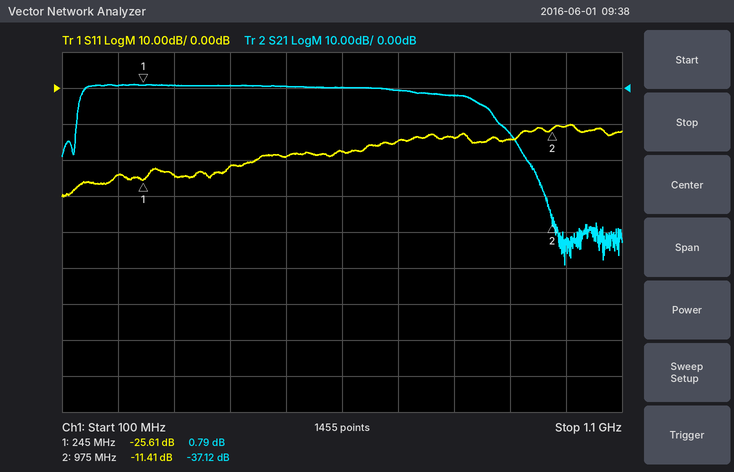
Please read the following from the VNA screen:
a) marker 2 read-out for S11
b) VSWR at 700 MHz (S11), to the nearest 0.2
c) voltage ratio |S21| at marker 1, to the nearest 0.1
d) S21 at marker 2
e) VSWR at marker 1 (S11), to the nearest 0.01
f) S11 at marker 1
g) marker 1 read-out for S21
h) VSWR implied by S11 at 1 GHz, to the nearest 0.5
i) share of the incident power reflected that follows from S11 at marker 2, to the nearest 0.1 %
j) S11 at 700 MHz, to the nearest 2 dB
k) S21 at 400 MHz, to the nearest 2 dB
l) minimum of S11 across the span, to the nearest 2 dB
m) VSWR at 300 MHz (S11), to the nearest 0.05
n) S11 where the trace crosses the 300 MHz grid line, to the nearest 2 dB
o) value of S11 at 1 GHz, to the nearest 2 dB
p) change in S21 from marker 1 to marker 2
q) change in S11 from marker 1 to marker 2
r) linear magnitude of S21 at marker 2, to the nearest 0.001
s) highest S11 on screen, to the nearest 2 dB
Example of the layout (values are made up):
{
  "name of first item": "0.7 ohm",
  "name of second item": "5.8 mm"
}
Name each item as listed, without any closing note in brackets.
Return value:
{
  "marker 2 read-out for S11": "-11.41 dB",
  "VSWR at 700 MHz (S11), to the nearest 0.2": "1.4",
  "voltage ratio |S21| at marker 1, to the nearest 0.1": "1.1",
  "S21 at marker 2": "-37.12 dB",
  "VSWR at marker 1 (S11), to the nearest 0.01": "1.11",
  "S11 at marker 1": "-25.61 dB",
  "marker 1 read-out for S21": "0.79 dB",
  "VSWR implied by S11 at 1 GHz, to the nearest 0.5": "2.0",
  "share of the incident power reflected that follows from S11 at marker 2, to the nearest 0.1 %": "7.2 %",
  "S11 at 700 MHz, to the nearest 2 dB": "-14 dB",
  "S21 at 400 MHz, to the nearest 2 dB": "0 dB",
  "minimum of S11 across the span, to the nearest 2 dB": "-30 dB",
  "VSWR at 300 MHz (S11), to the nearest 0.05": "1.15",
  "S11 where the trace crosses the 300 MHz grid line, to the nearest 2 dB": "-24 dB",
  "value of S11 at 1 GHz, to the nearest 2 dB": "-10 dB",
  "change in S21 from marker 1 to marker 2": "-37.91 dB",
  "change in S11 from marker 1 to marker 2": "14.20 dB",
  "linear magnitude of S21 at marker 2, to the nearest 0.001": "0.014",
  "highest S11 on screen, to the nearest 2 dB": "-10 dB"
}
